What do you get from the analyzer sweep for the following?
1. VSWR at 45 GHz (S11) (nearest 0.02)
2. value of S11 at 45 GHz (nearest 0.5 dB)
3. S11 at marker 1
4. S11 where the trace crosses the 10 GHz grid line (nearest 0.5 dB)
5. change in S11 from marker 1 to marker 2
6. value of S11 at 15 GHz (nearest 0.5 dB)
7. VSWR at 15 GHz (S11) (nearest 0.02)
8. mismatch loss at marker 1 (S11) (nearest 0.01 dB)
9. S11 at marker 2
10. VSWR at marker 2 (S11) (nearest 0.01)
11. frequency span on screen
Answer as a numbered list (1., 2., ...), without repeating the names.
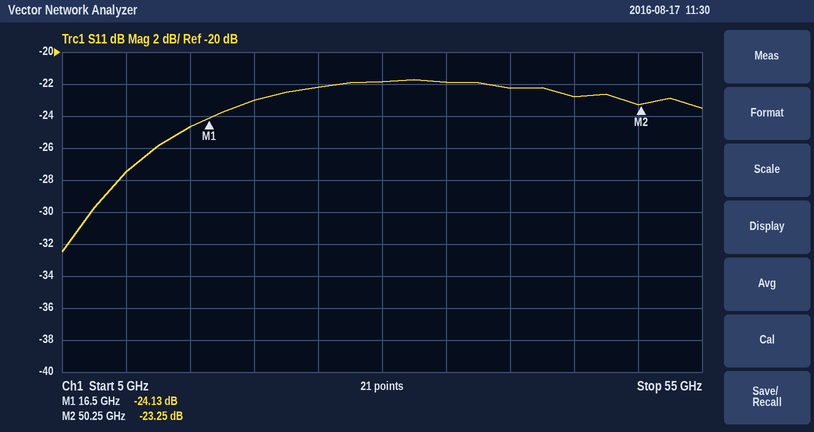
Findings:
1. 1.16
2. -23.0 dB
3. -24.13 dB
4. -27.5 dB
5. 0.88 dB
6. -24.5 dB
7. 1.12
8. 0.02 dB
9. -23.25 dB
10. 1.15
11. 50 GHz
